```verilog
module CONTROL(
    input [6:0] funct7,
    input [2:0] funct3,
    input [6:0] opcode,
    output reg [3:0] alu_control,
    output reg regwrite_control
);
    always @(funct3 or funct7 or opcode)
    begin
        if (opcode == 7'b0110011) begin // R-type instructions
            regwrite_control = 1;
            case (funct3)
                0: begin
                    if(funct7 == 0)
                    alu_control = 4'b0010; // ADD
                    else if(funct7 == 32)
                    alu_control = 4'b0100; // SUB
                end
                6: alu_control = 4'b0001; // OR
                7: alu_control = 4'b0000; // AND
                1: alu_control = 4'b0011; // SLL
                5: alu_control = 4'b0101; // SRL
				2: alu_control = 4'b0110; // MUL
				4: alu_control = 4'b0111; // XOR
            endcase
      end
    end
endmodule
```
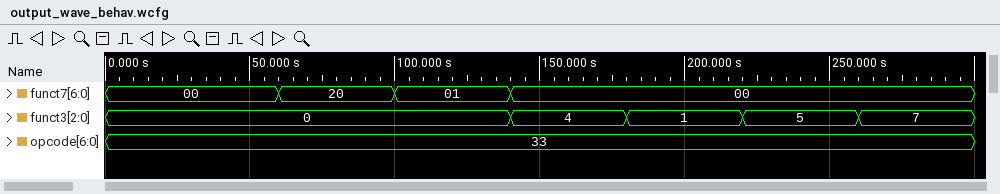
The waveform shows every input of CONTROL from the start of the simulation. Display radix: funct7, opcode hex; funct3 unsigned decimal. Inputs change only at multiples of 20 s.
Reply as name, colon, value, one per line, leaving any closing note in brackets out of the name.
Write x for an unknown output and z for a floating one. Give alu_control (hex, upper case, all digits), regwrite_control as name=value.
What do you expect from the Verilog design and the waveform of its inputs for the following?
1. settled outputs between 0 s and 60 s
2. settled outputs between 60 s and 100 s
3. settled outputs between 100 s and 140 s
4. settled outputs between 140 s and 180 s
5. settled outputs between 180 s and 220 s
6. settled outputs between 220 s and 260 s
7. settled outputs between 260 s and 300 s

settled outputs between 0 s and 60 s: alu_control=2, regwrite_control=1
settled outputs between 60 s and 100 s: alu_control=4, regwrite_control=1
settled outputs between 100 s and 140 s: alu_control=4, regwrite_control=1
settled outputs between 140 s and 180 s: alu_control=7, regwrite_control=1
settled outputs between 180 s and 220 s: alu_control=3, regwrite_control=1
settled outputs between 220 s and 260 s: alu_control=5, regwrite_control=1
settled outputs between 260 s and 300 s: alu_control=0, regwrite_control=1
